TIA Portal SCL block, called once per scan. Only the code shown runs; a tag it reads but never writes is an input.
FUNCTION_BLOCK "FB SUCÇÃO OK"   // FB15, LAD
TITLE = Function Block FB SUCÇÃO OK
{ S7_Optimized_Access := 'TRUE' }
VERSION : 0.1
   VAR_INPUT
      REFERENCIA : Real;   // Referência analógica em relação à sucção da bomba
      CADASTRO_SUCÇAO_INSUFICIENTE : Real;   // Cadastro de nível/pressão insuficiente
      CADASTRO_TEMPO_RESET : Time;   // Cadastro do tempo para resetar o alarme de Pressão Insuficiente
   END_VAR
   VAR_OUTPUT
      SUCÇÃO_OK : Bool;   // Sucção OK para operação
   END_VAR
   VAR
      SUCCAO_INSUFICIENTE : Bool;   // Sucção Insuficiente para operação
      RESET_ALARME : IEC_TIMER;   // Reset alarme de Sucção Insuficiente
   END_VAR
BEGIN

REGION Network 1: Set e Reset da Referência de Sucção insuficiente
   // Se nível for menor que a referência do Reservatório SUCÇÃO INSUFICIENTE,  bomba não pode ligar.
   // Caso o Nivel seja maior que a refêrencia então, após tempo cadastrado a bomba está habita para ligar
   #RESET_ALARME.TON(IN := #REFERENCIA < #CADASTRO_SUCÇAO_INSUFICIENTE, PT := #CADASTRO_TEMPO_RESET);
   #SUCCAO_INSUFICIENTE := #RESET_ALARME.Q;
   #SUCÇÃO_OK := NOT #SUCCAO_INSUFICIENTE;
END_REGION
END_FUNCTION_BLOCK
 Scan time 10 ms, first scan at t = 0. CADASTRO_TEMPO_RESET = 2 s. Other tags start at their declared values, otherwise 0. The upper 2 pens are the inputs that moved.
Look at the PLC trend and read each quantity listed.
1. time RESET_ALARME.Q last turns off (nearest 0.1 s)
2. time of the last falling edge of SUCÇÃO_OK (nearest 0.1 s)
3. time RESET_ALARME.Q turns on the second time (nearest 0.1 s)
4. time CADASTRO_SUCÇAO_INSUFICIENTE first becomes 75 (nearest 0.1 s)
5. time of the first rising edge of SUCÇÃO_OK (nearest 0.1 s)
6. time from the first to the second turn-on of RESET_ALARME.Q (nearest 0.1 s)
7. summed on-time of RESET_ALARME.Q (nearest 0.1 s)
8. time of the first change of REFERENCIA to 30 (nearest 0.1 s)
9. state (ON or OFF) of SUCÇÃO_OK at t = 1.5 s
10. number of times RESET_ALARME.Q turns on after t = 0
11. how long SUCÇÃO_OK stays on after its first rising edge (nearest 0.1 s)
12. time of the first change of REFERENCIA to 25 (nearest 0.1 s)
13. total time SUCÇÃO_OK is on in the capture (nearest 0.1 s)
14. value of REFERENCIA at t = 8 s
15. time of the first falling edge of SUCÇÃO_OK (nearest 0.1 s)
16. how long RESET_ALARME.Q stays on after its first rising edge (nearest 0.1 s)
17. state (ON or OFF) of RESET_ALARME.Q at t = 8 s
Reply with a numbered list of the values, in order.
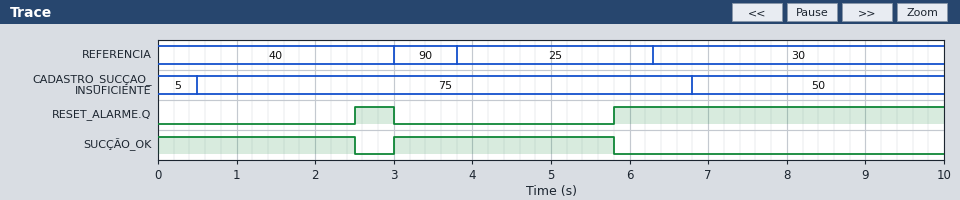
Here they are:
1. 3.0 s
2. 5.8 s
3. 5.8 s
4. 0.5 s
5. 3.0 s
6. 3.3 s
7. 4.7 s
8. 6.3 s
9. ON
10. 2
11. 2.8 s
12. 3.8 s
13. 5.3 s
14. 30
15. 2.5 s
16. 0.5 s
17. ON
